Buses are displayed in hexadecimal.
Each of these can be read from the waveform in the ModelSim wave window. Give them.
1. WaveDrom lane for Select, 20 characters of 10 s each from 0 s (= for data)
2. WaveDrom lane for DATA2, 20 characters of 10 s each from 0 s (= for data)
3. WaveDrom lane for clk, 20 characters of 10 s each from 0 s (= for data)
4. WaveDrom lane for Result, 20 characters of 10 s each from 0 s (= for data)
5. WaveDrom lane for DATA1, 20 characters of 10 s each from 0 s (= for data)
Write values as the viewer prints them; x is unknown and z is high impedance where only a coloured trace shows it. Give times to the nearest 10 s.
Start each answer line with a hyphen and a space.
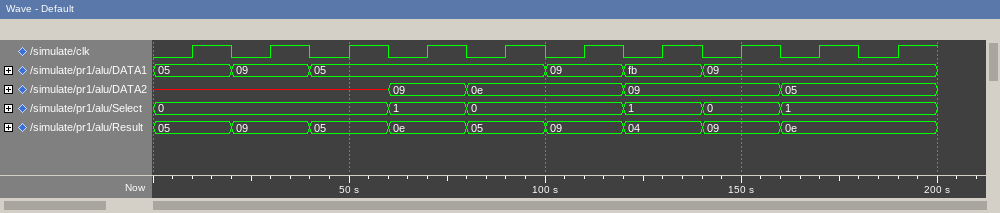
- {name: 'Select', wave: '=.....=.=...=.=.=...', data: '0 1 0 1 0 1'}
- {name: 'DATA2', wave: 'x.....=.=...=...=...', data: '09 0e 09 05'}
- {name: 'clk', wave: '01010101010101010101'}
- {name: 'Result', wave: '=.=.=.=.=.=.=.=.=...', data: '05 09 05 0e 05 09 04 09 0e'}
- {name: 'DATA1', wave: '=.=.=.....=.=.=.....', data: '05 09 05 09 fb 09'}
